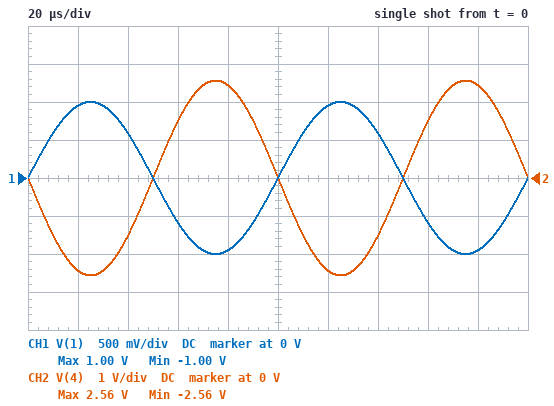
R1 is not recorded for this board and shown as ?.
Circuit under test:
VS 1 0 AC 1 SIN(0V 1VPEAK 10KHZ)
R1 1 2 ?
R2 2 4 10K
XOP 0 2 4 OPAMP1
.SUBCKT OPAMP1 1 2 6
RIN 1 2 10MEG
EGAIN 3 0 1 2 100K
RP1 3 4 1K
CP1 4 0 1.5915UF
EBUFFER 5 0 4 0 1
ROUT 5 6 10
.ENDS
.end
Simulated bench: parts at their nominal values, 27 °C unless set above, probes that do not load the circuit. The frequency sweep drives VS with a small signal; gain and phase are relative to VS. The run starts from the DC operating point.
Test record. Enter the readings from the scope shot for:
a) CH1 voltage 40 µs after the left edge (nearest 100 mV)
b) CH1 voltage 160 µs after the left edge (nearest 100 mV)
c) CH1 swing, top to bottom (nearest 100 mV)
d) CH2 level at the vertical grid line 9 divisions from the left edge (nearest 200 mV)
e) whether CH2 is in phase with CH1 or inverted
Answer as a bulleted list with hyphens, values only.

- 600 mV
- -600 mV
- 2.0 V
- 2.4 V
- inverted
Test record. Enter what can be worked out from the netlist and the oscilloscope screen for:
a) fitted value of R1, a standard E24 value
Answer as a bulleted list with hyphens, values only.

- 3.9 kΩ
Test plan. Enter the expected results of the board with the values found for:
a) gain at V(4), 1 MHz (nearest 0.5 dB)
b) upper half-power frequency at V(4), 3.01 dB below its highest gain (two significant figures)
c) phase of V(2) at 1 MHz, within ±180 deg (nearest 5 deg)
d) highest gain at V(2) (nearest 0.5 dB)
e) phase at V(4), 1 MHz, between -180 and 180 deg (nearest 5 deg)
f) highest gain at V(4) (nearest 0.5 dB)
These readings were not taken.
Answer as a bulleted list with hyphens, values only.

- 7.5 dB
- 2.8 MHz
- 70 deg
- -3.0 dB
- 160 deg
- 8.0 dB
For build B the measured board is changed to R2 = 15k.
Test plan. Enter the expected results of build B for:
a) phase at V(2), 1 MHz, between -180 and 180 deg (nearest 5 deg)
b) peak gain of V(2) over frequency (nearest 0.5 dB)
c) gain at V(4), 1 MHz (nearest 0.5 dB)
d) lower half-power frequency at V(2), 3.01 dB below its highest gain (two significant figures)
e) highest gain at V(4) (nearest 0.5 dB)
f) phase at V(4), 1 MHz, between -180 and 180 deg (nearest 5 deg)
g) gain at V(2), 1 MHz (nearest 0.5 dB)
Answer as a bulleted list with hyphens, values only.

- 65 deg
- -2.0 dB
- 11.0 dB
- 2.1 MHz
- 11.5 dB
- 155 deg
- -9.0 dB
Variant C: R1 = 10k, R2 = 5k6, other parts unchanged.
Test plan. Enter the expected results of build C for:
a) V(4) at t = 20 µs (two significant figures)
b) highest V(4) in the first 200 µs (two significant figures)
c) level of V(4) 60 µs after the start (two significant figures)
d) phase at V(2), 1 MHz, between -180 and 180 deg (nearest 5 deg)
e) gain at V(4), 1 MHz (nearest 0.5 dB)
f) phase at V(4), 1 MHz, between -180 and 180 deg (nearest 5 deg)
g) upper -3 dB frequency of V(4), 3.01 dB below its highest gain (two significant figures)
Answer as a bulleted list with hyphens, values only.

- -530 mV
- 560 mV
- 330 mV
- 80 deg
- -5.0 dB
- 170 deg
- 6.4 MHz
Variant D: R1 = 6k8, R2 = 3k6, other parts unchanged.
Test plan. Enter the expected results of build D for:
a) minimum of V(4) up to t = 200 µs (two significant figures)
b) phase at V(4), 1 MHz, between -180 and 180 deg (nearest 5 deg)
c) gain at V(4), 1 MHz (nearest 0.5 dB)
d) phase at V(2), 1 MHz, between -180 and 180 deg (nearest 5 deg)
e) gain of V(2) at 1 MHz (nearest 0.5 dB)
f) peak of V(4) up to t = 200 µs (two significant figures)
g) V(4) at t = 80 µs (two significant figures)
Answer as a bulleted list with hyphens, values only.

- -530 mV
- 170 deg
- -5.5 dB
- 80 deg
- -25.5 dB
- 530 mV
- 500 mV
